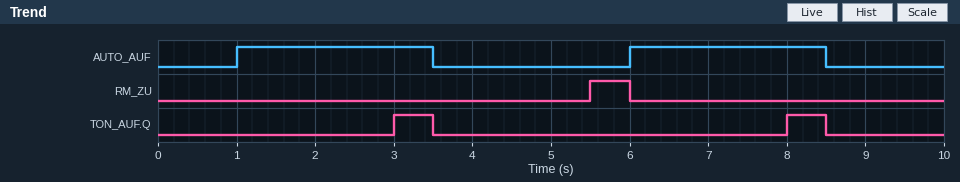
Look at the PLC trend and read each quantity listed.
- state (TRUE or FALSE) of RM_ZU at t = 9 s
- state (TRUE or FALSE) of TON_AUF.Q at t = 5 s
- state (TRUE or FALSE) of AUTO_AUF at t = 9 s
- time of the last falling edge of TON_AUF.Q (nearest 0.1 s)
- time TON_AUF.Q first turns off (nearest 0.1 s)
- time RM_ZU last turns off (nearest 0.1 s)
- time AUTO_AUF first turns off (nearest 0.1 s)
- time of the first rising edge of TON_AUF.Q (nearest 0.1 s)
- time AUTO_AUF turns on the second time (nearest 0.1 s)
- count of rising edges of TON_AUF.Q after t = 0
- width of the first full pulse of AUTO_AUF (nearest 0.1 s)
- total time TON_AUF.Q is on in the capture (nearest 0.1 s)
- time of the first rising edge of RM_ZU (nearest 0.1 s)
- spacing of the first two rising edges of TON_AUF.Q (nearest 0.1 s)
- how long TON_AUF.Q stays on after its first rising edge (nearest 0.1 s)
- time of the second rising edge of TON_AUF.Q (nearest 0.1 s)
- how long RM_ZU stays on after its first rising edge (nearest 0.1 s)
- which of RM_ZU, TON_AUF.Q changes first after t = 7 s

FALSE
FALSE
FALSE
8.5 s
3.5 s
6.0 s
3.5 s
3.0 s
6.0 s
2
2.5 s
1.0 s
5.5 s
5.0 s
0.5 s
8.0 s
0.5 s
TON_AUF.Q
